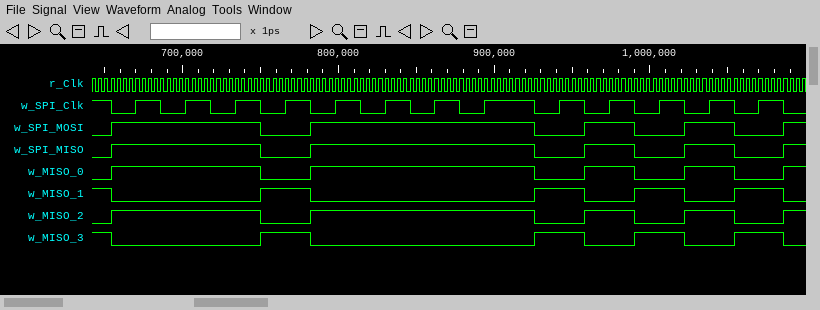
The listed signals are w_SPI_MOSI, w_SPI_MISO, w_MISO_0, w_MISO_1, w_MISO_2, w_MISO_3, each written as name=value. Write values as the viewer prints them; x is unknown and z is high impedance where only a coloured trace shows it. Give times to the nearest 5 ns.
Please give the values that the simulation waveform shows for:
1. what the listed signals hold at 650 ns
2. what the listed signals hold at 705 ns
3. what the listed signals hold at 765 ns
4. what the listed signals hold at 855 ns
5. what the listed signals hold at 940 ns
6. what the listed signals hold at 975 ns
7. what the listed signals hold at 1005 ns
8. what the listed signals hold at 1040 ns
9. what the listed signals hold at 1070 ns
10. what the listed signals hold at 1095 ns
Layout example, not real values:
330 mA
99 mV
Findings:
w_SPI_MOSI=0, w_SPI_MISO=0, w_MISO_0=0, w_MISO_1=1, w_MISO_2=0, w_MISO_3=1
w_SPI_MOSI=1, w_SPI_MISO=1, w_MISO_0=1, w_MISO_1=0, w_MISO_2=1, w_MISO_3=0
w_SPI_MOSI=0, w_SPI_MISO=0, w_MISO_0=0, w_MISO_1=1, w_MISO_2=0, w_MISO_3=1
w_SPI_MOSI=1, w_SPI_MISO=1, w_MISO_0=1, w_MISO_1=0, w_MISO_2=1, w_MISO_3=0
w_SPI_MOSI=0, w_SPI_MISO=0, w_MISO_0=0, w_MISO_1=1, w_MISO_2=0, w_MISO_3=1
w_SPI_MOSI=1, w_SPI_MISO=1, w_MISO_0=1, w_MISO_1=0, w_MISO_2=1, w_MISO_3=0
w_SPI_MOSI=0, w_SPI_MISO=0, w_MISO_0=0, w_MISO_1=1, w_MISO_2=0, w_MISO_3=1
w_SPI_MOSI=1, w_SPI_MISO=1, w_MISO_0=1, w_MISO_1=0, w_MISO_2=1, w_MISO_3=0
w_SPI_MOSI=0, w_SPI_MISO=0, w_MISO_0=0, w_MISO_1=1, w_MISO_2=0, w_MISO_3=1
w_SPI_MOSI=1, w_SPI_MISO=1, w_MISO_0=1, w_MISO_1=0, w_MISO_2=1, w_MISO_3=0
